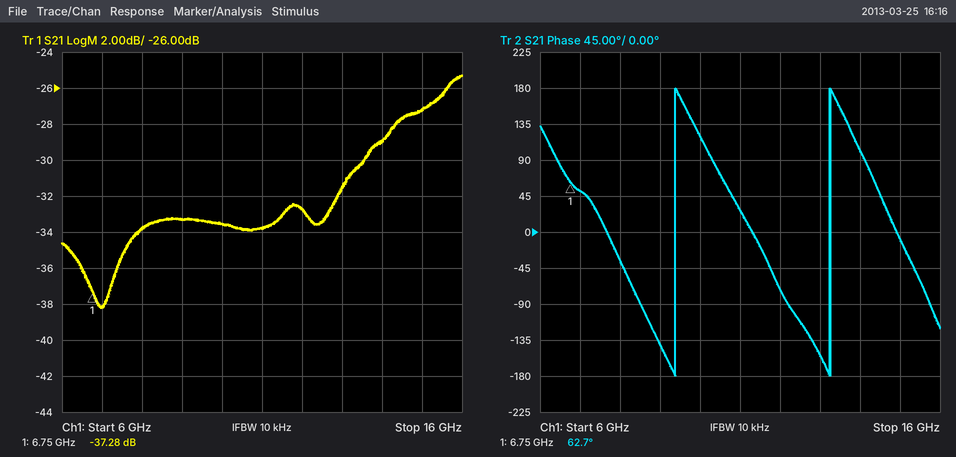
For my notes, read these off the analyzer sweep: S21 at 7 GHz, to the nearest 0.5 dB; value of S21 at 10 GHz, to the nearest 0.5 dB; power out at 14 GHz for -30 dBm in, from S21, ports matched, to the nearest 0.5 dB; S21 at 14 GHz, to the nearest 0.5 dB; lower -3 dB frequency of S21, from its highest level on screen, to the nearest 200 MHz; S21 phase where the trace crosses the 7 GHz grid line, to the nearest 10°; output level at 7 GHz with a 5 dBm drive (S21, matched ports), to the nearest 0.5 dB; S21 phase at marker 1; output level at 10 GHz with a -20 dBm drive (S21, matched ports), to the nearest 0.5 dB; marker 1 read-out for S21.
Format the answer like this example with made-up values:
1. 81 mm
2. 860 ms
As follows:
1. -38.0 dB
2. -33.5 dB
3. -59.0 dBm
4. -29.0 dB
5. 14.2 GHz
6. 50°
7. -33.0 dBm
8. 62.7°
9. -53.5 dBm
10. -37.28 dB
